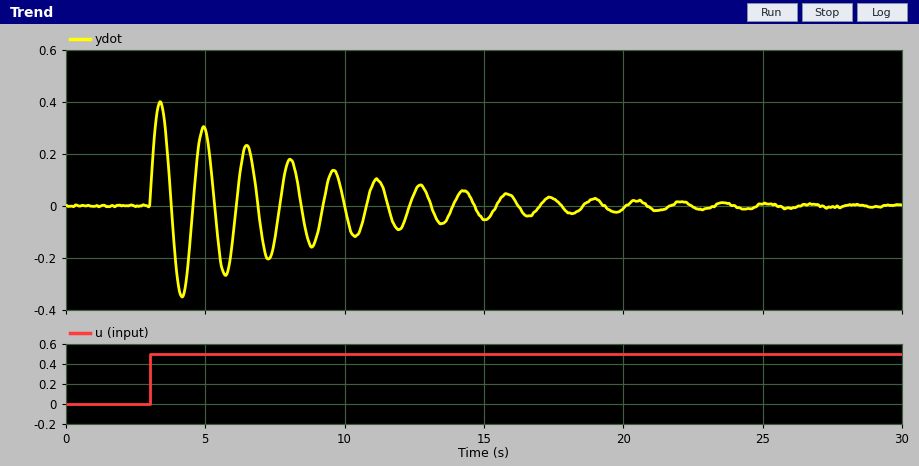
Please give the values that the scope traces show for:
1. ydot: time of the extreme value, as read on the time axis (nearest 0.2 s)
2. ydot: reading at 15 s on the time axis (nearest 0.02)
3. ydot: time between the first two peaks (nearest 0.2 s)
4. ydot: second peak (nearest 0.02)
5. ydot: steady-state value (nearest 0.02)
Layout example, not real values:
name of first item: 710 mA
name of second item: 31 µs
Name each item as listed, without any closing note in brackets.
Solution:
ydot: time of the extreme value, as read on the time axis: 3.4 s
ydot: reading at 15 s on the time axis: -0.06
ydot: time between the first two peaks: 1.6 s
ydot: second peak: 0.30
ydot: steady-state value: 0.00
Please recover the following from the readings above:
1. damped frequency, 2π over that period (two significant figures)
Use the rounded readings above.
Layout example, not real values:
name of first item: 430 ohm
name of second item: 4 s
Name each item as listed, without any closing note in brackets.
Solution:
damped frequency, 2π over that period: 3.9 rad/s
